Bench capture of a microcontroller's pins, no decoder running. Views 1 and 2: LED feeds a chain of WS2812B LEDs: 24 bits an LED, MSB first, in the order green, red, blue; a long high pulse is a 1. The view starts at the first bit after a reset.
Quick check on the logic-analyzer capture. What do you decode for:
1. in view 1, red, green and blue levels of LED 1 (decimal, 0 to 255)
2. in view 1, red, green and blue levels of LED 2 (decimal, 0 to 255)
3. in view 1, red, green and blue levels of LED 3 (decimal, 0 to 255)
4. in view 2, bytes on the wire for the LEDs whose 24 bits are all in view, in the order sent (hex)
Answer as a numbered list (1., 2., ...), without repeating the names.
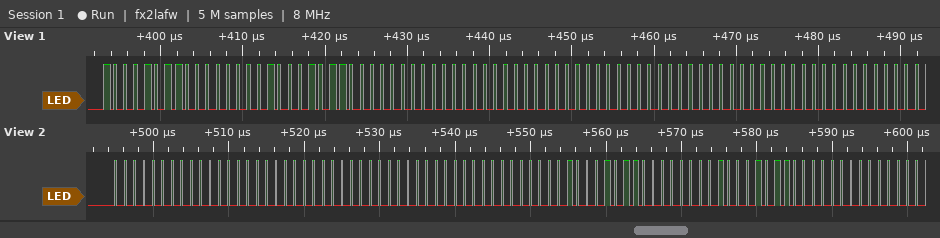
1. 0, 139, 139
2. 0, 0, 0
3. 0, 0, 0
4. 00 00 00 00 00 00 8B 00 8B
